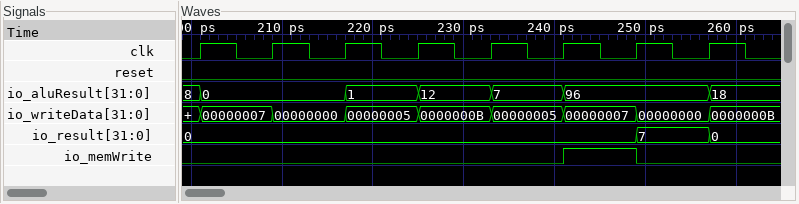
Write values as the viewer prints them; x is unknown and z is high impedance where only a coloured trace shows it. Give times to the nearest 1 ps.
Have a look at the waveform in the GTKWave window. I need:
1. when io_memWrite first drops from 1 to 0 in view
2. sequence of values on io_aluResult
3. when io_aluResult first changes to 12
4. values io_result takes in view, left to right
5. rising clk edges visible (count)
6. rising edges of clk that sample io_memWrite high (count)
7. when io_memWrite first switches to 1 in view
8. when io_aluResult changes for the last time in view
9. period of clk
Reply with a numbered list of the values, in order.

1. 249 ps
2. 8, 0, 1, 12, 7, 96, 18
3. 225 ps
4. 0, 7, 0
5. 8
6. 1
7. 241 ps
8. 257 ps
9. 8 ps
